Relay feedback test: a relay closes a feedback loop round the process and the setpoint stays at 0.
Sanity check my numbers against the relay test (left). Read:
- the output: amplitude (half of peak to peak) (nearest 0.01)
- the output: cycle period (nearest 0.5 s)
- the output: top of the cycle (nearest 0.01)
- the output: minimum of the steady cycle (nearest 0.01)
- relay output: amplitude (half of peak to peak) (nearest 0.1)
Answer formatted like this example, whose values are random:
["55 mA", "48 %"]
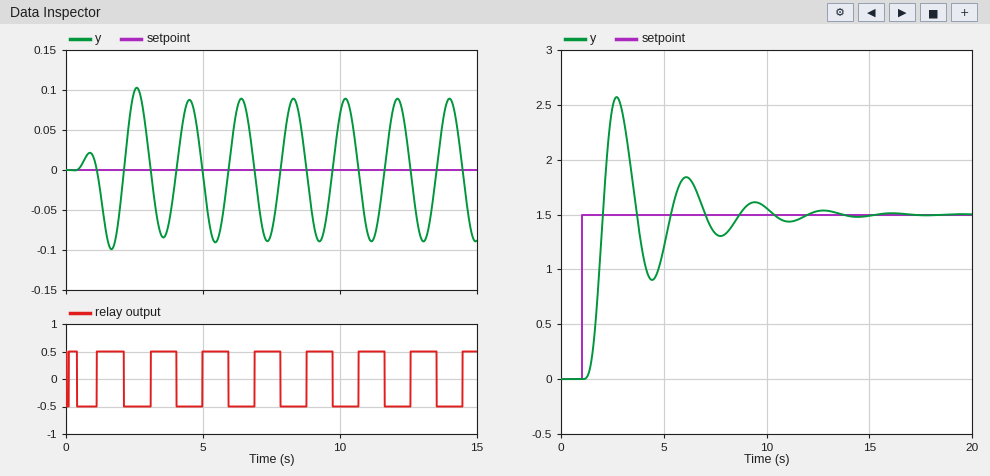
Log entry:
["0.09", "2.0 s", "0.09", "-0.09", "0.5"]
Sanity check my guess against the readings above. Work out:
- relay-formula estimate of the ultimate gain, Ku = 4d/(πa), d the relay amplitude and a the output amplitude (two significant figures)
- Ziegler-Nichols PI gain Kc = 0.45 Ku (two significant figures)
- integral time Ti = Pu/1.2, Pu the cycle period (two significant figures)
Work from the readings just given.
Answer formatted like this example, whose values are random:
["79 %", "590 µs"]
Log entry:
["7.1", "3.2", "1.7 s"]
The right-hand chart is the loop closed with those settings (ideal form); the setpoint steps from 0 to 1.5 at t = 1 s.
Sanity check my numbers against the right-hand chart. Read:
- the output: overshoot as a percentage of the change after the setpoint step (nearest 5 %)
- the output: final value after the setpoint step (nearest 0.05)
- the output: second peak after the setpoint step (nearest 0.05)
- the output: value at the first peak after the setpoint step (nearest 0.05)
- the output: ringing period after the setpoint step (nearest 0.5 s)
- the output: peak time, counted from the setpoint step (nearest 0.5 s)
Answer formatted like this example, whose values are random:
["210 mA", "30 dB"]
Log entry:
["70 %", "1.50", "1.85", "2.55", "3.5 s", "1.5 s"]
